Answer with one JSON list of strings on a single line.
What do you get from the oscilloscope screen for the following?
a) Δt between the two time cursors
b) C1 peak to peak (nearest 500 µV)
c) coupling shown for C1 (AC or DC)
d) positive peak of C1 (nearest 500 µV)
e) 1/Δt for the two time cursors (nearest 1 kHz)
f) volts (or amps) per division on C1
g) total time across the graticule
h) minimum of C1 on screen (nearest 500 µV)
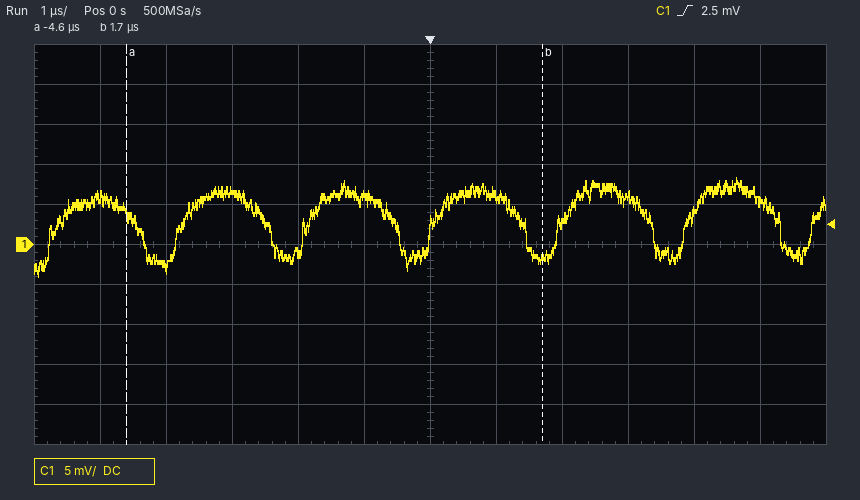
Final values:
["6.3 µs", "12.5 mV", "DC", "8.5 mV", "159 kHz", "5 mV", "12 µs", "-4.0 mV"]
